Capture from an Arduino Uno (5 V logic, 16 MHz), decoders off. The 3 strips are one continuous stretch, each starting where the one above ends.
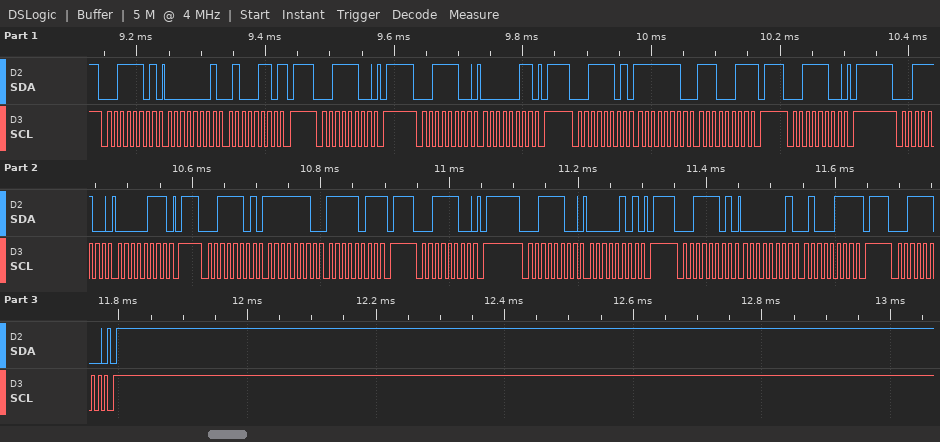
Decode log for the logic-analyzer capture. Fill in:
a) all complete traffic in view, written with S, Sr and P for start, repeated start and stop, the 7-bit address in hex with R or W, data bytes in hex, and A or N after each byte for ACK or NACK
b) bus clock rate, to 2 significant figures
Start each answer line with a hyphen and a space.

- S 1ER A 01 A 46 N P S 1EW A P S 1EW A 03 A P S 1ER A FE A E3 N P S 1EW A P S 1EW A 07 A P S 1ER A FE A FB N P S 1EW A P S 1EW A 05 A P S 1ER A 01 A 47 N P S 1EW A P
- 100 kHz
